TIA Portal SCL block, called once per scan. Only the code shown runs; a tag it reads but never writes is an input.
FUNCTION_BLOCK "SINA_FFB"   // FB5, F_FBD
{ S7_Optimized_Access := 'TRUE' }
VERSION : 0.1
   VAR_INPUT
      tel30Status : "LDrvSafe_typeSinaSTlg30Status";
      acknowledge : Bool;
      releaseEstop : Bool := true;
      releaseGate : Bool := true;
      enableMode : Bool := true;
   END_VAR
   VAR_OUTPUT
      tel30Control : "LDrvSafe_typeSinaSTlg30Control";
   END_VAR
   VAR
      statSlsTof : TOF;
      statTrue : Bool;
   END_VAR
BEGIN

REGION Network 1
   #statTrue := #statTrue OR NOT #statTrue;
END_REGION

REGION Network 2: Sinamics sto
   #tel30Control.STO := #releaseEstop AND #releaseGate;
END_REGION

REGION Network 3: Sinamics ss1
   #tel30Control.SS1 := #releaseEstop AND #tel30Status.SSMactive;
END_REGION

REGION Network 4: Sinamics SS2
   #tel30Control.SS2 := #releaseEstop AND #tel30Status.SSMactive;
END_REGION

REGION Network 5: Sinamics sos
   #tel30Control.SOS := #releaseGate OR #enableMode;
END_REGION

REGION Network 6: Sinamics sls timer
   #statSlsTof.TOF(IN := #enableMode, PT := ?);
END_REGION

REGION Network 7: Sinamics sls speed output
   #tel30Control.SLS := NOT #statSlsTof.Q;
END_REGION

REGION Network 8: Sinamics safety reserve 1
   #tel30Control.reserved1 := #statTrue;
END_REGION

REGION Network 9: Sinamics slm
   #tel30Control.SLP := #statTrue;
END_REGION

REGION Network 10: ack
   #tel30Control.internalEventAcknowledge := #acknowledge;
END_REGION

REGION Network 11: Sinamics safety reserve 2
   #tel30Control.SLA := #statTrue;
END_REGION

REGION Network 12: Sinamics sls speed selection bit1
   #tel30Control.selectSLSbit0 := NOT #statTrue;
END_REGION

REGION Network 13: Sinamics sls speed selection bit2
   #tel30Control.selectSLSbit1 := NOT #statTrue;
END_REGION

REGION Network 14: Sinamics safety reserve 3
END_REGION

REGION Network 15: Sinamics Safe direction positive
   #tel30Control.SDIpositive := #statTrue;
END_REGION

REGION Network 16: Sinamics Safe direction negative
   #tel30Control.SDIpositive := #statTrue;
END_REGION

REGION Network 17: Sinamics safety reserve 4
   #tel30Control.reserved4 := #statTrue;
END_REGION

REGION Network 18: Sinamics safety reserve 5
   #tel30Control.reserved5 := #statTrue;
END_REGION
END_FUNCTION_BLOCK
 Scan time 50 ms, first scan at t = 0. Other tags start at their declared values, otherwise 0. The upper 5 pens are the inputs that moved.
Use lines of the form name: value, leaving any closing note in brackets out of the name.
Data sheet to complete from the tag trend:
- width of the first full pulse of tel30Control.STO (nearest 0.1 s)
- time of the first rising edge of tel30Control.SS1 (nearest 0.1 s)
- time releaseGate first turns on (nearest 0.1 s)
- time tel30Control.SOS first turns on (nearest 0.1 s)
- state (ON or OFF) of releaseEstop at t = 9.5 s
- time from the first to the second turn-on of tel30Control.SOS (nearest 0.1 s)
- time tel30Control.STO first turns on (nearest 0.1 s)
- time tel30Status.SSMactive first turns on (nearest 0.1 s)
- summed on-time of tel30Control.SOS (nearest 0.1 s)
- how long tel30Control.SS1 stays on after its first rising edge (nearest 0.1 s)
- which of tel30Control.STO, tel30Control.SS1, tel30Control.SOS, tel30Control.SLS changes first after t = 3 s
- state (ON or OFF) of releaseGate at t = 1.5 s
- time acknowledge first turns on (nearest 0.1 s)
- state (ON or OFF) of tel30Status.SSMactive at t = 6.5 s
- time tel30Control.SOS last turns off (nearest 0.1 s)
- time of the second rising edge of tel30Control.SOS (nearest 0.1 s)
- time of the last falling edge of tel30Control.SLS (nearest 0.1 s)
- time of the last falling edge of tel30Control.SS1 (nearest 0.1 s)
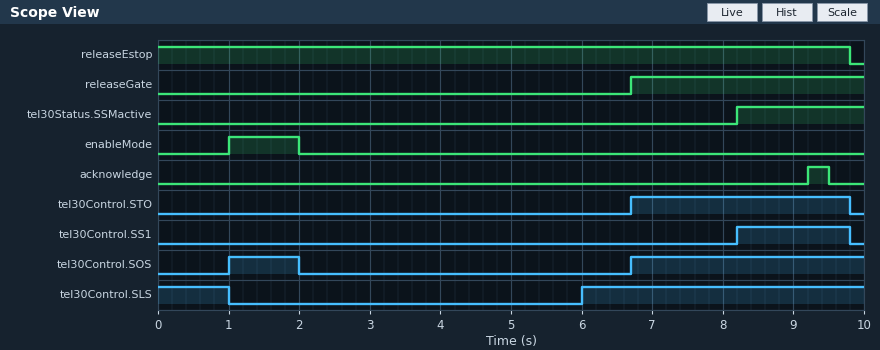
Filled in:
width of the first full pulse of tel30Control.STO: 3.1 s
time of the first rising edge of tel30Control.SS1: 8.2 s
time releaseGate first turns on: 6.7 s
time tel30Control.SOS first turns on: 1.0 s
state (ON or OFF) of releaseEstop at t = 9.5 s: ON
time from the first to the second turn-on of tel30Control.SOS: 5.7 s
time tel30Control.STO first turns on: 6.7 s
time tel30Status.SSMactive first turns on: 8.2 s
summed on-time of tel30Control.SOS: 4.3 s
how long tel30Control.SS1 stays on after its first rising edge: 1.6 s
which of tel30Control.STO, tel30Control.SS1, tel30Control.SOS, tel30Control.SLS changes first after t = 3 s: tel30Control.SLS
state (ON or OFF) of releaseGate at t = 1.5 s: OFF
time acknowledge first turns on: 9.2 s
state (ON or OFF) of tel30Status.SSMactive at t = 6.5 s: OFF
time tel30Control.SOS last turns off: 2.0 s
time of the second rising edge of tel30Control.SOS: 6.7 s
time of the last falling edge of tel30Control.SLS: 1.0 s
time of the last falling edge of tel30Control.SS1: 9.8 s
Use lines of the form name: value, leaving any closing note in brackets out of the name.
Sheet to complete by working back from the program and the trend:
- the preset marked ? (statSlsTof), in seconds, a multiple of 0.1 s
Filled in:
the preset marked ? (statSlsTof), in seconds, a multiple of 0.1 s: 4.0 s
